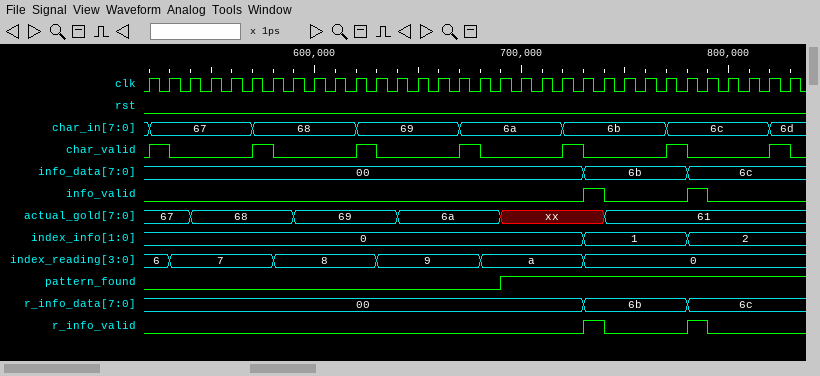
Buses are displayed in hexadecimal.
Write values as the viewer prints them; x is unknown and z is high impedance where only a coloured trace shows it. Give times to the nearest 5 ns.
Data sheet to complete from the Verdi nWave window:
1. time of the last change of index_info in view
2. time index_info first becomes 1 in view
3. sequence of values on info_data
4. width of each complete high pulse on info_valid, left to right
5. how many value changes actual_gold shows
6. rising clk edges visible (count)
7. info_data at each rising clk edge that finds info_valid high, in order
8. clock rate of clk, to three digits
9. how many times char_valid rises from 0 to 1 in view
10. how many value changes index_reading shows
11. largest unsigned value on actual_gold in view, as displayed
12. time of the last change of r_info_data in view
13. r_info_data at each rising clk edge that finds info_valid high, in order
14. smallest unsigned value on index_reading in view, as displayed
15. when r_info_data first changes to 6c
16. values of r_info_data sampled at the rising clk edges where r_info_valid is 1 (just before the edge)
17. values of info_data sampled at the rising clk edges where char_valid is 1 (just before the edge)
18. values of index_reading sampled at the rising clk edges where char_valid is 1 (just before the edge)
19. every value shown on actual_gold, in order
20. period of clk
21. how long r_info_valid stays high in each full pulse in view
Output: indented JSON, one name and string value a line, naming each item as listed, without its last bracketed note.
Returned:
{
  "time of the last change of index_info in view": "780 ns",
  "time index_info first becomes 1 in view": "730 ns",
  "sequence of values on info_data": "00, 6b, 6c",
  "width of each complete high pulse on info_valid, left to right": "10 ns, 10 ns",
  "how many value changes actual_gold shows": "5",
  "rising clk edges visible": "32",
  "info_data at each rising clk edge that finds info_valid high, in order": "6b, 6c",
  "clock rate of clk, to three digits": "100 MHz",
  "how many times char_valid rises from 0 to 1 in view": "7",
  "how many value changes index_reading shows": "5",
  "largest unsigned value on actual_gold in view, as displayed": "6a",
  "time of the last change of r_info_data in view": "780 ns",
  "r_info_data at each rising clk edge that finds info_valid high, in order": "6b, 6c",
  "smallest unsigned value on index_reading in view, as displayed": "0",
  "when r_info_data first changes to 6c": "780 ns",
  "values of r_info_data sampled at the rising clk edges where r_info_valid is 1": "6b, 6c",
  "values of info_data sampled at the rising clk edges where char_valid is 1": "00, 00, 00, 00, 00, 6b, 6c",
  "values of index_reading sampled at the rising clk edges where char_valid is 1": "6, 7, 8, 9, a, 0, 0",
  "every value shown on actual_gold, in order": "67, 68, 69, 6a, xx, 61",
  "period of clk": "10 ns",
  "how long r_info_valid stays high in each full pulse in view": "10 ns, 10 ns"
}
